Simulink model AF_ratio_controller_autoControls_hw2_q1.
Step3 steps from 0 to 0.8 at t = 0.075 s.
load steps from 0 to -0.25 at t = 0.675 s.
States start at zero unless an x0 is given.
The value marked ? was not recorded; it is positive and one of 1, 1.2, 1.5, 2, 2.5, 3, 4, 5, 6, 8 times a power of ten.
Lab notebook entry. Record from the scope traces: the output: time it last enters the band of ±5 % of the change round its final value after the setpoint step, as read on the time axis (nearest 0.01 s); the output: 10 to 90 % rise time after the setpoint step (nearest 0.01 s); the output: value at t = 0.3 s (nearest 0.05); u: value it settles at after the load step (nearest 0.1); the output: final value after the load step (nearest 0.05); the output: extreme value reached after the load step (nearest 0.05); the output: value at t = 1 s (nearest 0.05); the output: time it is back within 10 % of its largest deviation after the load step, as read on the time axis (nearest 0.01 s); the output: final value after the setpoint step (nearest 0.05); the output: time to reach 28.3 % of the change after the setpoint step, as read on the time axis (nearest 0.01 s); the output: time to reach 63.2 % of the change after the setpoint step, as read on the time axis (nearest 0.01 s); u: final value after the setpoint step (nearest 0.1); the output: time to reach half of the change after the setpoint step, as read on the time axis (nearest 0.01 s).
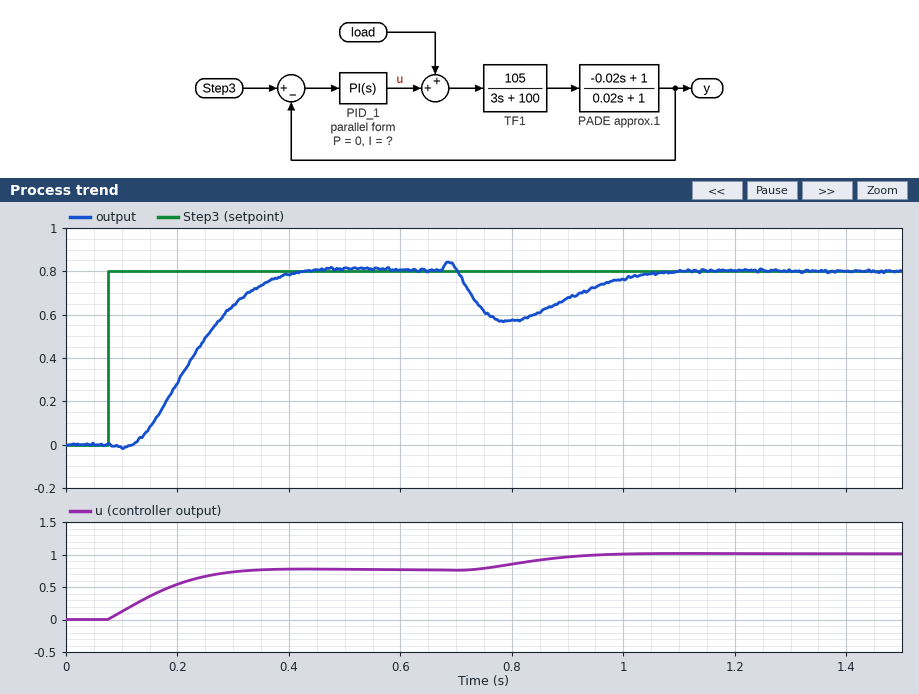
0.37 s
0.19 s
0.65
1.0
0.80
0.55
0.75
1.02 s
0.80
0.19 s
0.25 s
0.8
0.23 s
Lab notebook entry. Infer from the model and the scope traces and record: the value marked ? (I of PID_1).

6
